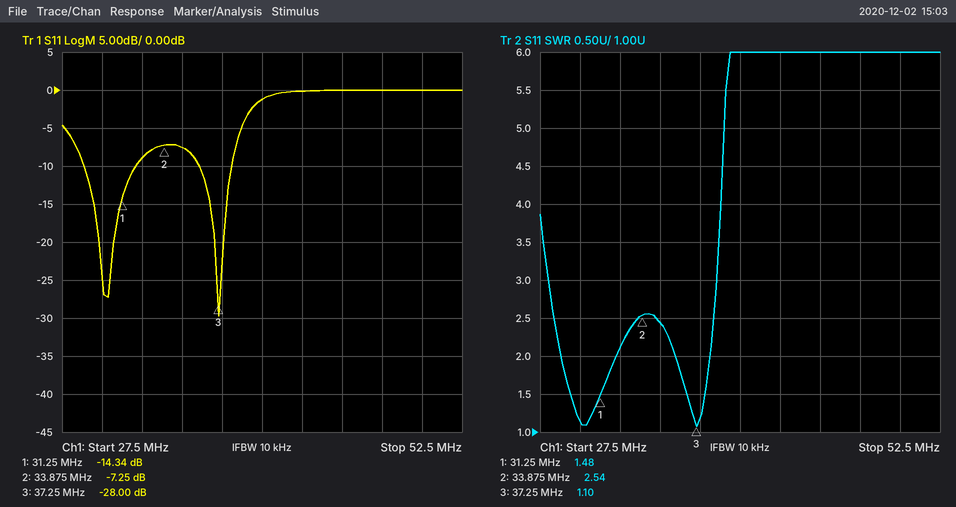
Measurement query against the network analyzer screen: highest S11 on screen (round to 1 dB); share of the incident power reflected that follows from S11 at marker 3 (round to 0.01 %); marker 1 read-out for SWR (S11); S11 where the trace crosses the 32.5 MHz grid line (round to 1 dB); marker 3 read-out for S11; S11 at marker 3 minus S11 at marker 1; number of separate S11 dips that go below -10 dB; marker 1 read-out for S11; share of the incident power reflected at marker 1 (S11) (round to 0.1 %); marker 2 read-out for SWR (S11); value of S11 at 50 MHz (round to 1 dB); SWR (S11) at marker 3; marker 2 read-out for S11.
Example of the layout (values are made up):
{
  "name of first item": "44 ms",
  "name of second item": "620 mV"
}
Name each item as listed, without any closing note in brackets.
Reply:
{
  "highest S11 on screen": "0 dB",
  "share of the incident power reflected that follows from S11 at marker 3": "0.16 %",
  "marker 1 read-out for SWR": "1.48",
  "S11 where the trace crosses the 32.5 MHz grid line": "-9 dB",
  "marker 3 read-out for S11": "-28.00 dB",
  "S11 at marker 3 minus S11 at marker 1": "-13.66 dB",
  "number of separate S11 dips that go below -10 dB": "2",
  "marker 1 read-out for S11": "-14.34 dB",
  "share of the incident power reflected at marker 1 (S11)": "3.7 %",
  "marker 2 read-out for SWR": "2.54",
  "value of S11 at 50 MHz": "0 dB",
  "SWR (S11) at marker 3": "1.10",
  "marker 2 read-out for S11": "-7.25 dB"
}
